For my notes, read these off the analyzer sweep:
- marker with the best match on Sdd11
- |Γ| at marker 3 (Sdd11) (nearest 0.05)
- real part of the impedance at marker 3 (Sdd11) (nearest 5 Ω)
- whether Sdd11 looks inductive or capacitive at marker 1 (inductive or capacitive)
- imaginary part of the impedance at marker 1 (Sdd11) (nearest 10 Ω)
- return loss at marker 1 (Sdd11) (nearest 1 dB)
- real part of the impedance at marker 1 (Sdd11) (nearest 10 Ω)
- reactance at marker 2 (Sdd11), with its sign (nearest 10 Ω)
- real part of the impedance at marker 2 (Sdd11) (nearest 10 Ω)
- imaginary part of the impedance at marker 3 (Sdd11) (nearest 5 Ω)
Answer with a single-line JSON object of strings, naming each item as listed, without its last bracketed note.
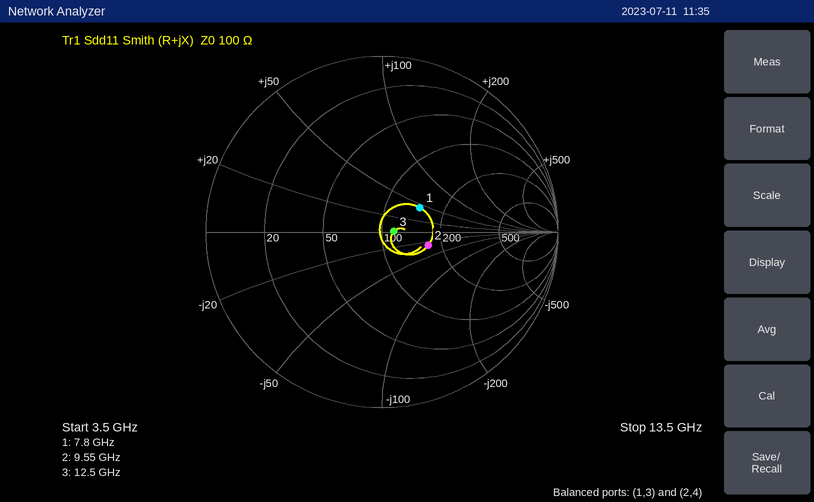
{"marker with the best match on Sdd11": "marker 3", "|Γ| at marker 3 (Sdd11)": "0.05", "real part of the impedance at marker 3 (Sdd11)": "115 Ω", "whether Sdd11 looks inductive or capacitive at marker 1": "inductive", "imaginary part of the impedance at marker 1 (Sdd11)": "+40 Ω", "return loss at marker 1 (Sdd11)": "12 dB", "real part of the impedance at marker 1 (Sdd11)": "150 Ω", "reactance at marker 2 (Sdd11), with its sign": "-30 Ω", "real part of the impedance at marker 2 (Sdd11)": "170 Ω", "imaginary part of the impedance at marker 3 (Sdd11)": "0 Ω"}
